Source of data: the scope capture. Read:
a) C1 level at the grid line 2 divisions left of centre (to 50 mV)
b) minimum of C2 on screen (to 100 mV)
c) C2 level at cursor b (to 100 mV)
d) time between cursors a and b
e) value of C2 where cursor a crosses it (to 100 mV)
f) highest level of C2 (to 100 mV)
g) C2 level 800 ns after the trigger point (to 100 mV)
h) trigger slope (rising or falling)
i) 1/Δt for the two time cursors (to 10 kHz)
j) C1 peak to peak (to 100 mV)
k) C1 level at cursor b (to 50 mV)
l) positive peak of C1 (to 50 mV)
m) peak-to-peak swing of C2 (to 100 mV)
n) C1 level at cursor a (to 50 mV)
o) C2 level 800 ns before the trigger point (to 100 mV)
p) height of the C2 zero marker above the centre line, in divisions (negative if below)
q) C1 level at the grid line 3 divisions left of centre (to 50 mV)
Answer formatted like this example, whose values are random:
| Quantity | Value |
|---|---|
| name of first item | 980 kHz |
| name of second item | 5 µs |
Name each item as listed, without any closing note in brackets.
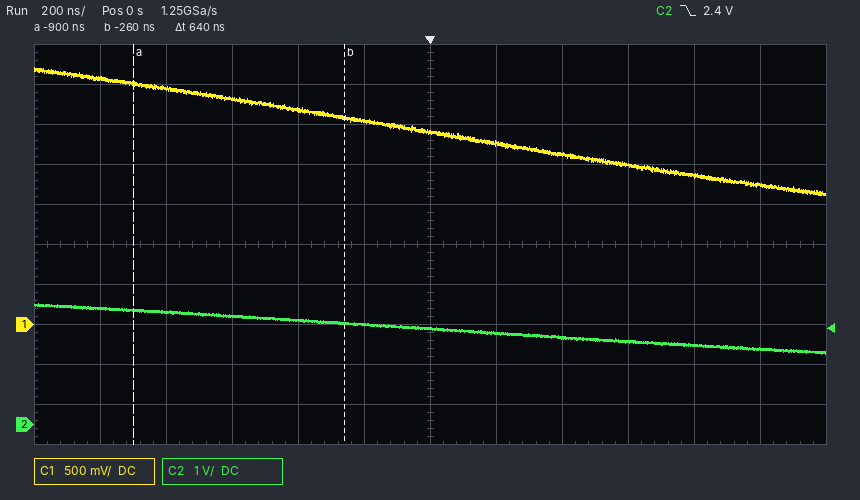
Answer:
| Quantity | Value |
|---|---|
| C1 level at the grid line 2 divisions left of centre | 2.70 V |
| minimum of C2 on screen | 1.8 V |
| C2 level at cursor b | 2.5 V |
| time between cursors a and b | 640 ns |
| value of C2 where cursor a crosses it | 2.9 V |
| highest level of C2 | 3.0 V |
| C2 level 800 ns after the trigger point | 2.0 V |
| trigger slope | falling |
| 1/Δt for the two time cursors | 1.56 MHz |
| C1 peak to peak | 1.60 V |
| C1 level at cursor b | 2.60 V |
| positive peak of C1 | 3.20 V |
| peak-to-peak swing of C2 | 1.2 V |
| C1 level at cursor a | 3.00 V |
| C2 level 800 ns before the trigger point | 2.8 V |
| height of the C2 zero marker above the centre line, in divisions | -4.5 div |
| C1 level at the grid line 3 divisions left of centre | 2.85 V |
